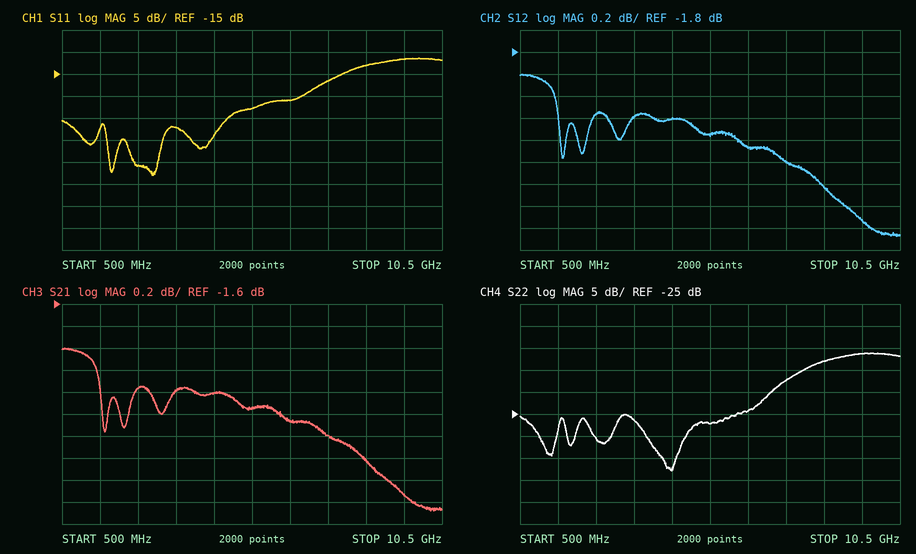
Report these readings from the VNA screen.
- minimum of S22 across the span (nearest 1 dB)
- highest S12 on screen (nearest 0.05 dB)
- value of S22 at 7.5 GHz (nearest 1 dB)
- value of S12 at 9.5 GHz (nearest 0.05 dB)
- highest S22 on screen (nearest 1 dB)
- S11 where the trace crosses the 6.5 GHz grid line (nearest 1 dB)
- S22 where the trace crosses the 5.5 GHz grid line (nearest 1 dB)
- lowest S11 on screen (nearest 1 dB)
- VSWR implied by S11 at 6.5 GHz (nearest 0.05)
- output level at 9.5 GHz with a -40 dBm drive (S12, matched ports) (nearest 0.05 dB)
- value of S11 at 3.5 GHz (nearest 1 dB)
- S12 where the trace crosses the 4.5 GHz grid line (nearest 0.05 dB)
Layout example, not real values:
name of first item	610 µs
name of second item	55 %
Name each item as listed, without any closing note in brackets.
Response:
minimum of S22 across the span	-38 dB
highest S12 on screen	-2.00 dB
value of S22 at 7.5 GHz	-17 dB
value of S12 at 9.5 GHz	-3.35 dB
highest S22 on screen	-11 dB
S11 where the trace crosses the 6.5 GHz grid line	-21 dB
S22 where the trace crosses the 5.5 GHz grid line	-27 dB
lowest S11 on screen	-38 dB
VSWR implied by S11 at 6.5 GHz	1.20
output level at 9.5 GHz with a -40 dBm drive (S12, matched ports)	-43.35 dBm
value of S11 at 3.5 GHz	-27 dB
S12 where the trace crosses the 4.5 GHz grid line	-2.40 dB
